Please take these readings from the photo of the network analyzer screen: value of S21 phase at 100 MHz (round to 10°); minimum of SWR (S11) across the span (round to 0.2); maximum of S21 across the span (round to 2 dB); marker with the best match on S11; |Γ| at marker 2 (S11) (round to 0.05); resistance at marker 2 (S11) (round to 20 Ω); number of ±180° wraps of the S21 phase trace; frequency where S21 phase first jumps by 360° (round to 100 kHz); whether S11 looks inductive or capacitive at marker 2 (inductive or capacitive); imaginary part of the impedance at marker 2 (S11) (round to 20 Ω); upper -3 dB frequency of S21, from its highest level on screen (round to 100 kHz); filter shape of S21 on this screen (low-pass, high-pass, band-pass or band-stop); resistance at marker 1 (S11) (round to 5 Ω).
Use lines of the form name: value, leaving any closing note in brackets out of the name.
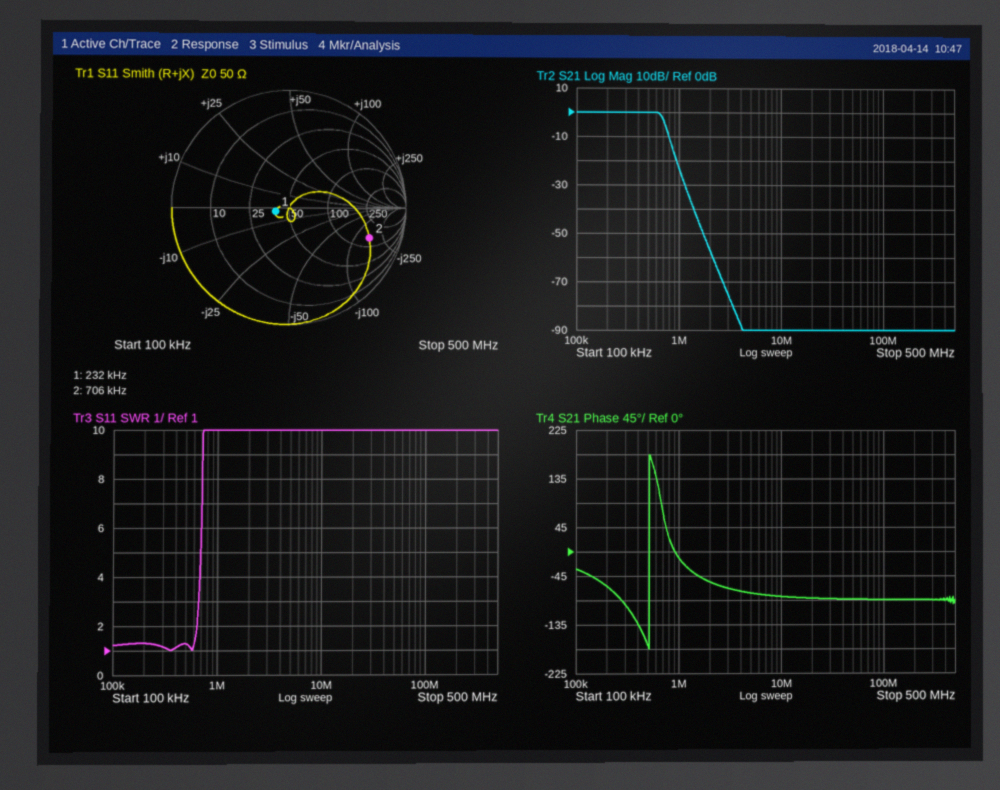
value of S21 phase at 100 MHz: -90°
minimum of SWR (S11) across the span: 1.0
maximum of S21 across the span: 0 dB
marker with the best match on S11: marker 1
|Γ| at marker 2 (S11): 0.75
resistance at marker 2 (S11): 140 Ω
number of ±180° wraps of the S21 phase trace: 1
frequency where S21 phase first jumps by 360°: 500 kHz
whether S11 looks inductive or capacitive at marker 2: capacitive
imaginary part of the impedance at marker 2 (S11): -160 Ω
upper -3 dB frequency of S21, from its highest level on screen: 700 kHz
filter shape of S21 on this screen: low-pass
resistance at marker 1 (S11): 40 Ω
